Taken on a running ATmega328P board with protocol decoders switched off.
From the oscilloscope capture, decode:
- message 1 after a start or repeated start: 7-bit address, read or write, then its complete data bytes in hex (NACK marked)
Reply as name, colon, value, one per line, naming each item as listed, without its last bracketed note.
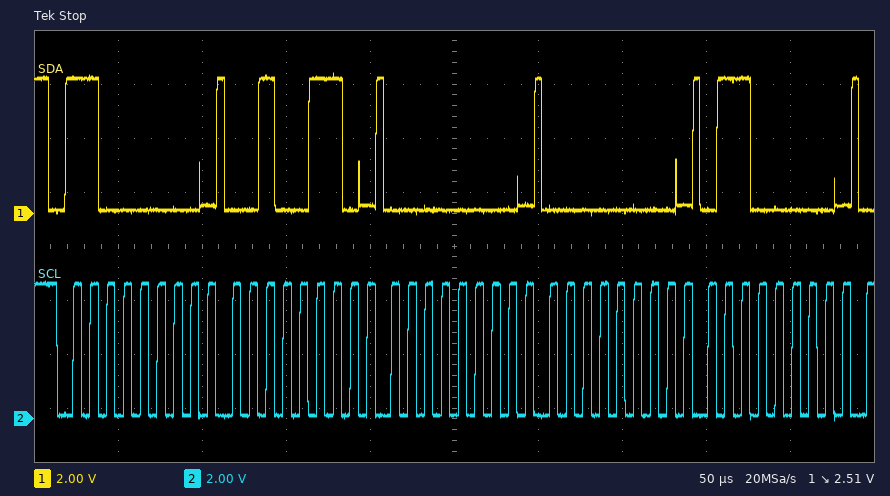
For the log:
message 1 after a start or repeated start: 7-bit address, read or write, then its complete data bytes in hex: 0x60 write: 26 00 00 60
